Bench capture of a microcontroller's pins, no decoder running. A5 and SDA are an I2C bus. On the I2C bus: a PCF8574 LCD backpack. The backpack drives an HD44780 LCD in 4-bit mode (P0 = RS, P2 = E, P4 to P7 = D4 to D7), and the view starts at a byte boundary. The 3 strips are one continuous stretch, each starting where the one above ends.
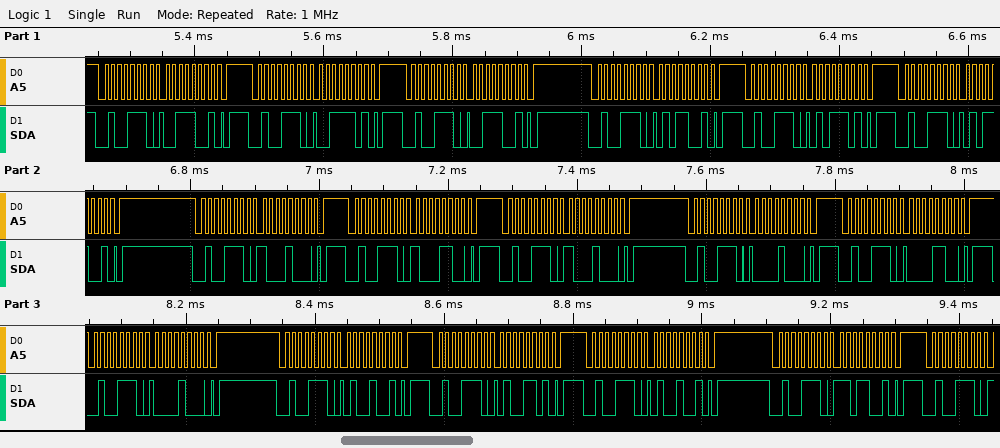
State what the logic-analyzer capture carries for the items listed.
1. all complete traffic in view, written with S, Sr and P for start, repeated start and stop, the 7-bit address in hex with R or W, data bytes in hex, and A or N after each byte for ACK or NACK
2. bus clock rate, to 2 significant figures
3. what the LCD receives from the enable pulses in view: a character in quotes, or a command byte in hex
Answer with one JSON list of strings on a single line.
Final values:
["S 27W A 39 A P S 27W A 3D A P S 27W A 39 A P S 27W A 59 A P S 27W A 5D A P S 27W A 59 A P S 27W A 88 A P S 27W A 8C A P S 27W A 88 A P S 27W A 08 A P S 27W A 0C A P S 27W A 08 A P S 27W A 49 A P S 27W A 4D A P S 27W A 49 A P S 27W A D9 A P S 27W A", "100 kHz", "'5' 0x80"]
